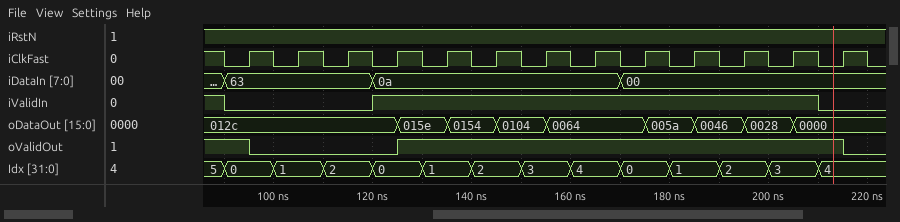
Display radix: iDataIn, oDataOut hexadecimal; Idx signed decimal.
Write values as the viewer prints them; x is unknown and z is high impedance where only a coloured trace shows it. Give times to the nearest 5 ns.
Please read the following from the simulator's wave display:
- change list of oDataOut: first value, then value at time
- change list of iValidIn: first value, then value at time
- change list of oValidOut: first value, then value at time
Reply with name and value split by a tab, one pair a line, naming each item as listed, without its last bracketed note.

change list of oDataOut: first value, then value at time	012c, 015e at 125 ns, 0154 at 135 ns, 0104 at 145 ns, 0064 at 155 ns, 005a at 175 ns, 0046 at 185 ns, 0028 at 195 ns, 0000 at 205 ns
change list of iValidIn: first value, then value at time	1, 0 at 90 ns, 1 at 120 ns, 0 at 210 ns
change list of oValidOut: first value, then value at time	1, 0 at 95 ns, 1 at 125 ns, 0 at 215 ns
